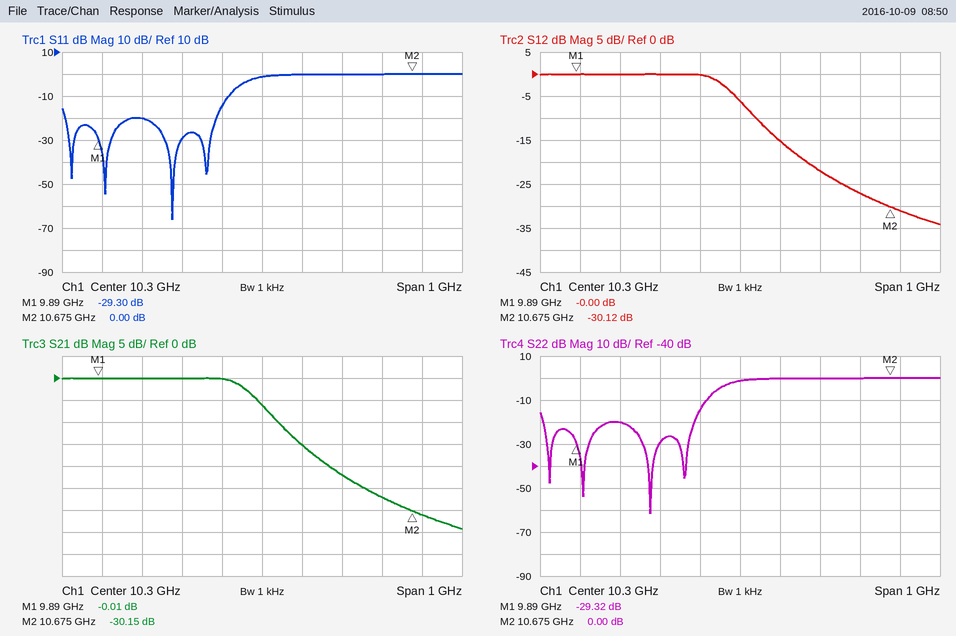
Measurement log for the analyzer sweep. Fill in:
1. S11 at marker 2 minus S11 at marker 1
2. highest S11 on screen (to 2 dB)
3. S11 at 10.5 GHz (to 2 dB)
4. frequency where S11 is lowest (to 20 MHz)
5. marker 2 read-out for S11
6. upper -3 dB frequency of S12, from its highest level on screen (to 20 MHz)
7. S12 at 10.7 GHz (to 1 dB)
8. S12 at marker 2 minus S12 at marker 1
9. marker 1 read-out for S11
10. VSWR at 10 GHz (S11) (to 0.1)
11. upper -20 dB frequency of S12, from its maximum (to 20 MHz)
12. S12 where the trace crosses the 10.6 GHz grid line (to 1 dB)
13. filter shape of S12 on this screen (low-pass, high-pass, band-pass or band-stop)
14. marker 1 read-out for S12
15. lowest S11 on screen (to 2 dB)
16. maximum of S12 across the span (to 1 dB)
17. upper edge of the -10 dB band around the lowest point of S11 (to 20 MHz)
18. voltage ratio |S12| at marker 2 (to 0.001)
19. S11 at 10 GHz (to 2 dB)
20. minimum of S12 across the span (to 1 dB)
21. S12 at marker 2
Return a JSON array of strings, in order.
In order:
["29.30 dB", "0 dB", "0 dB", "10.08 GHz", "0.00 dB", "10.26 GHz", "-31 dB", "-30.12 dB", "-29.30 dB", "1.2", "10.46 GHz", "-27 dB", "low-pass", "-0.00 dB", "-66 dB", "0 dB", "10.22 GHz", "0.031", "-20 dB", "-34 dB", "-30.12 dB"]
